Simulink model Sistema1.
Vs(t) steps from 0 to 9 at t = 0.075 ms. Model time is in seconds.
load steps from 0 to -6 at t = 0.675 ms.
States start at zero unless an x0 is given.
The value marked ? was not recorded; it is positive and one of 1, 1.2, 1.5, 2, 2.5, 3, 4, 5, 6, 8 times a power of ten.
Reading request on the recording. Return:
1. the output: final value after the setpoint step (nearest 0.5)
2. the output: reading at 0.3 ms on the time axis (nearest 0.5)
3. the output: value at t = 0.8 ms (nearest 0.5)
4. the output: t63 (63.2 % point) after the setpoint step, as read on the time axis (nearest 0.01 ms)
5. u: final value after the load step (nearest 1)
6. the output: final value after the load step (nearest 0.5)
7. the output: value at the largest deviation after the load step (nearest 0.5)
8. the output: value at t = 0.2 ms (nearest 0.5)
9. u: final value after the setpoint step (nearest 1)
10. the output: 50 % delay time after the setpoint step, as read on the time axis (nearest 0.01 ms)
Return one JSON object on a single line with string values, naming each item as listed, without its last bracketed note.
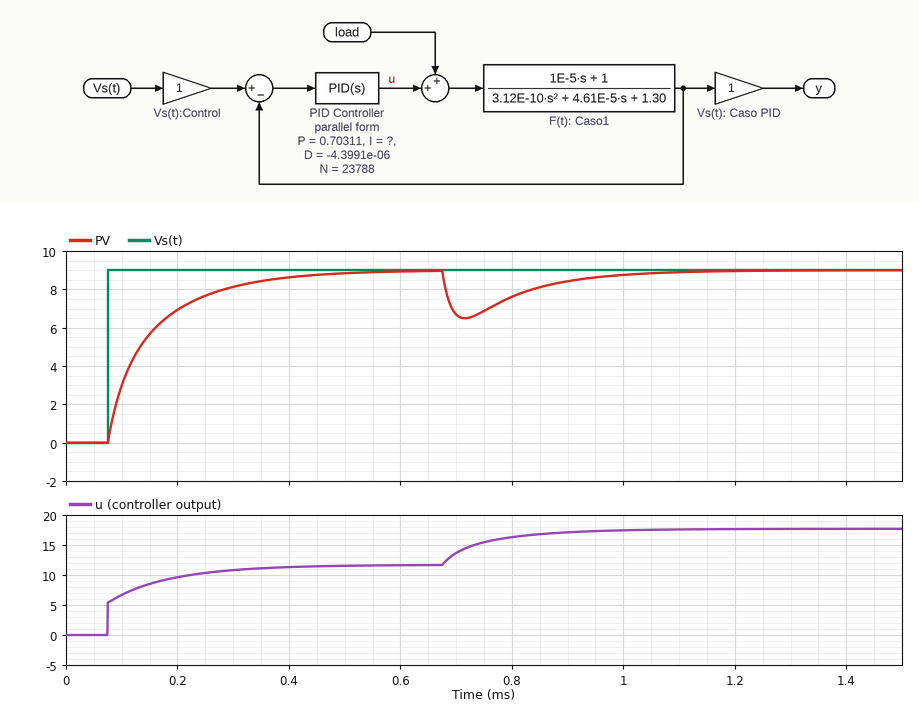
{"the output: final value after the setpoint step": "9.0", "the output: reading at 0.3 ms on the time axis": "8.0", "the output: value at t = 0.8 ms": "7.5", "the output: t63 (63.2 % point) after the setpoint step, as read on the time axis": "0.15 ms", "u: final value after the load step": "18", "the output: final value after the load step": "9.0", "the output: value at the largest deviation after the load step": "6.5", "the output: value at t = 0.2 ms": "7.0", "u: final value after the setpoint step": "12", "the output: 50 % delay time after the setpoint step, as read on the time axis": "0.12 ms"}
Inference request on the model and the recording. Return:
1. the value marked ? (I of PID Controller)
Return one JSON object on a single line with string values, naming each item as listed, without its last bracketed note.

{"the value marked ?": "15000"}
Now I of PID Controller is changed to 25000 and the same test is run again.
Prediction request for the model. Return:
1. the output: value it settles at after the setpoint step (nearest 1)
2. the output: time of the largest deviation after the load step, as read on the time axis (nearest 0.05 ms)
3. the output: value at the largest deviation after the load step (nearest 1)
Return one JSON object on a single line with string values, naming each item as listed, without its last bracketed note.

{"the output: value it settles at after the setpoint step": "9", "the output: time of the largest deviation after the load step, as read on the time axis": "0.70 ms", "the output: value at the largest deviation after the load step": "7"}
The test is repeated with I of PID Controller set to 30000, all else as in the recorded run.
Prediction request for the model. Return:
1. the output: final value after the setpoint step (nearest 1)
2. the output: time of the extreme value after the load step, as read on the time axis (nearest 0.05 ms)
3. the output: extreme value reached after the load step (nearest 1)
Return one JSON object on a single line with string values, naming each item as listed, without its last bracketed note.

{"the output: final value after the setpoint step": "9", "the output: time of the extreme value after the load step, as read on the time axis": "0.70 ms", "the output: extreme value reached after the load step": "7"}
